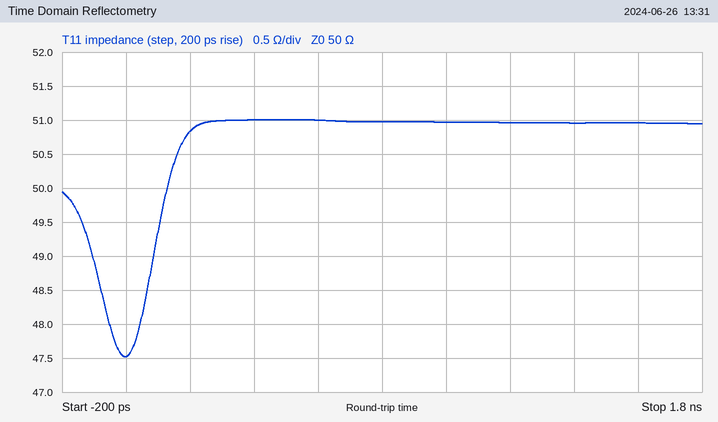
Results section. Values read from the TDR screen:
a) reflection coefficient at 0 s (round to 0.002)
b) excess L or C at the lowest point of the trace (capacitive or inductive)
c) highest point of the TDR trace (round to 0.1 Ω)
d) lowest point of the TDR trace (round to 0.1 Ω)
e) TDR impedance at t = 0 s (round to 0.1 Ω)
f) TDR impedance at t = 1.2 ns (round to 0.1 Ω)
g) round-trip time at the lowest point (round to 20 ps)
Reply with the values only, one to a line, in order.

-0.026
capacitive
51.0 Ω
47.5 Ω
47.5 Ω
51.0 Ω
0 ps
